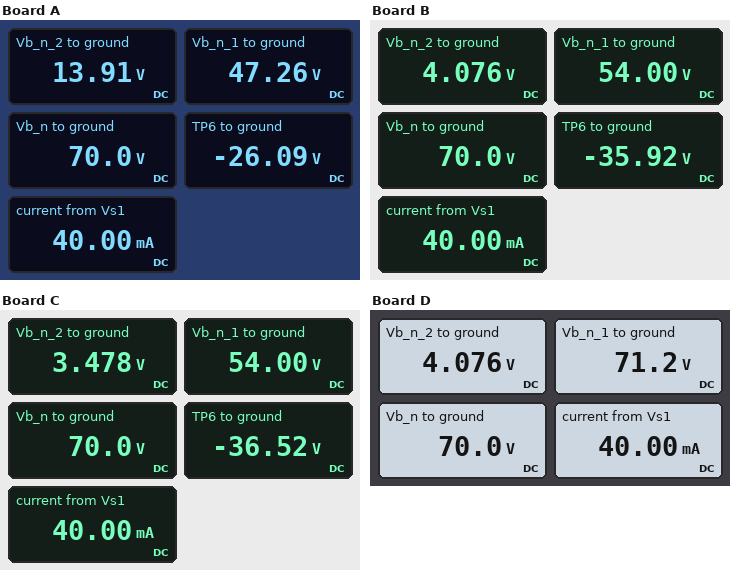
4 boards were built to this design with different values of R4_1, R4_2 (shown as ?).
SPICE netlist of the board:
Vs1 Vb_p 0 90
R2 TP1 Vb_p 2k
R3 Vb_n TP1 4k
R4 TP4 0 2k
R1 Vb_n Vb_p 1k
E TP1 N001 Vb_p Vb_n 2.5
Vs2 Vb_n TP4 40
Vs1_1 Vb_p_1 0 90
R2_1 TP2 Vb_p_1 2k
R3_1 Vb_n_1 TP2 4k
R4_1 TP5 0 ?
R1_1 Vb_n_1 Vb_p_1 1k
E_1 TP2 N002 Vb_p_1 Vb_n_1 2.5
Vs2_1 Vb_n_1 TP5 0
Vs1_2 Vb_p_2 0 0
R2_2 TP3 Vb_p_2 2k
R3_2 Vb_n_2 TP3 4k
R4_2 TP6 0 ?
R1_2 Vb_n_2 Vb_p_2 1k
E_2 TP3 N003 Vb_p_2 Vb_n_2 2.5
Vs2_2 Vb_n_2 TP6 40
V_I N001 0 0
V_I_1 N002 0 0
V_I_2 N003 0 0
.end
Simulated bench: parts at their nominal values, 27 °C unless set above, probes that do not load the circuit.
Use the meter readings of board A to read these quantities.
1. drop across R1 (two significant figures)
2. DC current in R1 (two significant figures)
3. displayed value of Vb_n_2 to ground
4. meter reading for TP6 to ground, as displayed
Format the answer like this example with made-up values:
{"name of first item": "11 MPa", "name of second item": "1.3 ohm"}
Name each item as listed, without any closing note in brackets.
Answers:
{"drop across R1": "20 V", "DC current in R1": "20 mA", "displayed value of Vb_n_2 to ground": "13.91 V", "meter reading for TP6 to ground, as displayed": "-26.09 V"}
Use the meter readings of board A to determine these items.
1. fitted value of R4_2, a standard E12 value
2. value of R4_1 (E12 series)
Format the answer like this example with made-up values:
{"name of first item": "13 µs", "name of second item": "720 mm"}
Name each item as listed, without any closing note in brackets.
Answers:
{"fitted value of R4_2, a standard E12 value": "1 kΩ", "value of R4_1": "820 Ω"}
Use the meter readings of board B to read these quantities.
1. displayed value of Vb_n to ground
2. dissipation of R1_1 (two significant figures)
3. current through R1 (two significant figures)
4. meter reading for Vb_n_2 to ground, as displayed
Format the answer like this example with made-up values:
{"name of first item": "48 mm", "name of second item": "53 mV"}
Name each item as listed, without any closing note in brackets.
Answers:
{"displayed value of Vb_n to ground": "70.0 V", "dissipation of R1_1": "1.3 W", "current through R1": "20 mA", "meter reading for Vb_n_2 to ground, as displayed": "4.076 V"}
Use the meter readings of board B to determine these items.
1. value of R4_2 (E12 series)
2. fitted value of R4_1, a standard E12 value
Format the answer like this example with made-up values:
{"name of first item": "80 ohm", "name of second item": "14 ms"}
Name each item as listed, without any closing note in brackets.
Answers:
{"value of R4_2": "4.7 kΩ", "fitted value of R4_1, a standard E12 value": "1.2 kΩ"}
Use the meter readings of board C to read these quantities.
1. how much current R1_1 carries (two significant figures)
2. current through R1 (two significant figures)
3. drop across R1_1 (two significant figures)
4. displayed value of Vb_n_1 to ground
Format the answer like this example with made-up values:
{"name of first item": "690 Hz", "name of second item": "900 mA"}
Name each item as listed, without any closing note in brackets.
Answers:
{"how much current R1_1 carries": "36 mA", "current through R1": "20 mA", "drop across R1_1": "36 V", "displayed value of Vb_n_1 to ground": "54.00 V"}
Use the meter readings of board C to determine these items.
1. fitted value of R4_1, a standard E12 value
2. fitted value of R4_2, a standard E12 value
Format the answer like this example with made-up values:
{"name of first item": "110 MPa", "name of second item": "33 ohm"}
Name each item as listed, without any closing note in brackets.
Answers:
{"fitted value of R4_1, a standard E12 value": "1.2 kΩ", "fitted value of R4_2, a standard E12 value": "5.6 kΩ"}
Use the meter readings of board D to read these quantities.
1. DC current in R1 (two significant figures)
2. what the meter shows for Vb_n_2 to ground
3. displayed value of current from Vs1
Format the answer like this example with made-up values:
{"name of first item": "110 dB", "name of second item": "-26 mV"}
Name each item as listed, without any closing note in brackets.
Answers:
{"DC current in R1": "20 mA", "what the meter shows for Vb_n_2 to ground": "4.076 V", "displayed value of current from Vs1": "40.00 mA"}
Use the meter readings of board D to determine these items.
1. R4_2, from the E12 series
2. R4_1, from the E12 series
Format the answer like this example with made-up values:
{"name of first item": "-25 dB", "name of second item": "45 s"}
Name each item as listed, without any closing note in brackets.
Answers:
{"R4_2, from the E12 series": "4.7 kΩ", "R4_1, from the E12 series": "5.6 kΩ"}
